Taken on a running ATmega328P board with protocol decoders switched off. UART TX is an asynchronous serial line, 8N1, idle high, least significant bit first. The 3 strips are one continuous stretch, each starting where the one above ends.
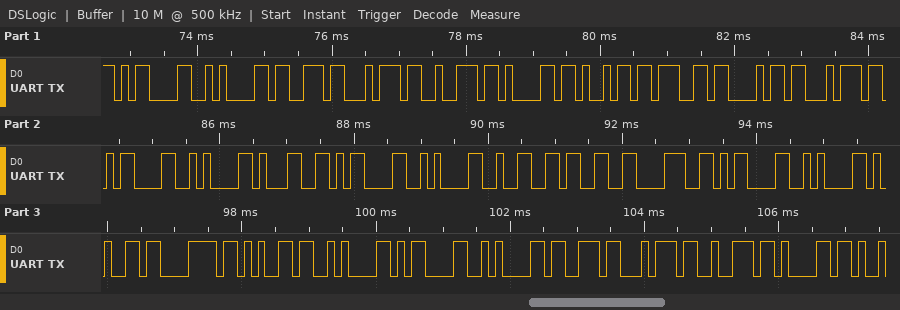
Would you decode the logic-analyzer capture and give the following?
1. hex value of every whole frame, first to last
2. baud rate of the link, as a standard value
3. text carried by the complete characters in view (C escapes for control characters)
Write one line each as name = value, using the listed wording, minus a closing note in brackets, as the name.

hex value of every whole frame, first to last = 0x0D 0x0A 0x73 0x74 0x72 0x61 0x69 0x67 0x68 0x74 0x0D 0x0A 0x31 0x0D 0x0A 0x32 0x33 0x38 0x0D 0x0A 0x65 0x78 0x65 0x0A 0x0D 0x0A 0x73 0x74 0x72 0x61
baud rate of the link, as a standard value = 9600 baud
text carried by the complete characters in view = "\r\nstraight\r\n1\r\n238\r\nexe\n\r\nstra"
